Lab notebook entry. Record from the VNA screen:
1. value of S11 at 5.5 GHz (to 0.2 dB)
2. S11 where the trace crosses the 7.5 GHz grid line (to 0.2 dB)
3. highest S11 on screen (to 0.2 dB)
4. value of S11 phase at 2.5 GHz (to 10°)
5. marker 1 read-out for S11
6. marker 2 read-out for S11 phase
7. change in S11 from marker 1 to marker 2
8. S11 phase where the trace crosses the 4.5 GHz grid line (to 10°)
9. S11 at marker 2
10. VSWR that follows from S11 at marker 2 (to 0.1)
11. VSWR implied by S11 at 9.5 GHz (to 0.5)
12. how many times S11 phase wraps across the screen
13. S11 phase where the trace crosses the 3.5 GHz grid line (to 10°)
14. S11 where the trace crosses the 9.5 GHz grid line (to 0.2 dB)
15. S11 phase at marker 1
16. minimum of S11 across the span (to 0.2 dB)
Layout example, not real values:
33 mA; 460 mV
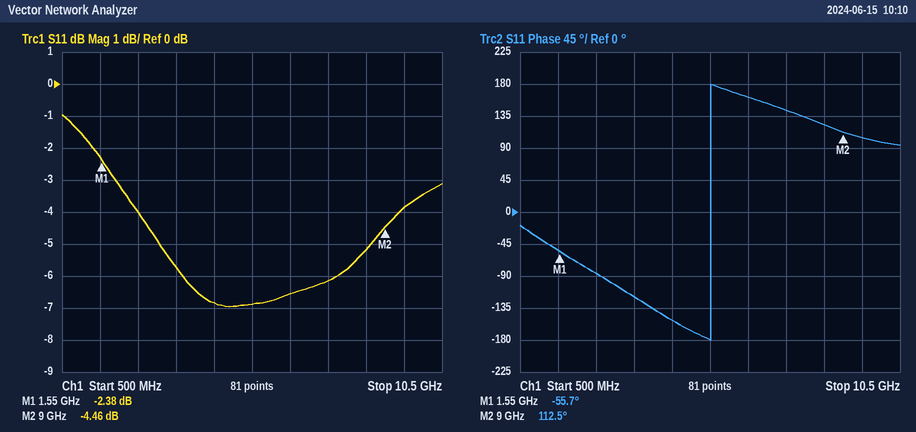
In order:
-6.8 dB; -6.2 dB; -1.0 dB; -90°; -2.38 dB; 112.5°; -2.08 dB; -150°; -4.46 dB; 4.0; 4.5; 1; -120°; -3.8 dB; -55.7°; -7.0 dB
